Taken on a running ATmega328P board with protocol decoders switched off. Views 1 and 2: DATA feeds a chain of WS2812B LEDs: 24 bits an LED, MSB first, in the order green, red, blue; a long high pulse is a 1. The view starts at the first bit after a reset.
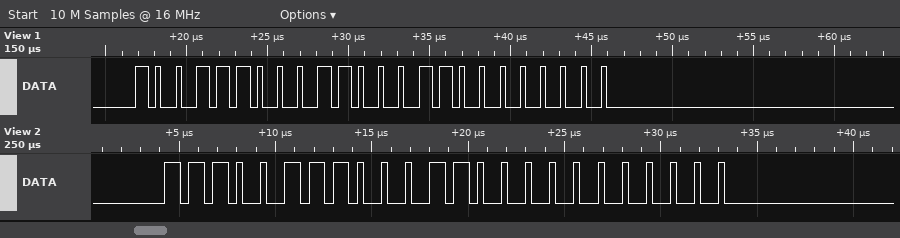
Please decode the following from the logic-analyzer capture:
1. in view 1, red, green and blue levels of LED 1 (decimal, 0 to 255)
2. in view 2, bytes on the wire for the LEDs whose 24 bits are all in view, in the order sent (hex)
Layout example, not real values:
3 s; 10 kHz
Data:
99, 156, 0; E7 18 00
